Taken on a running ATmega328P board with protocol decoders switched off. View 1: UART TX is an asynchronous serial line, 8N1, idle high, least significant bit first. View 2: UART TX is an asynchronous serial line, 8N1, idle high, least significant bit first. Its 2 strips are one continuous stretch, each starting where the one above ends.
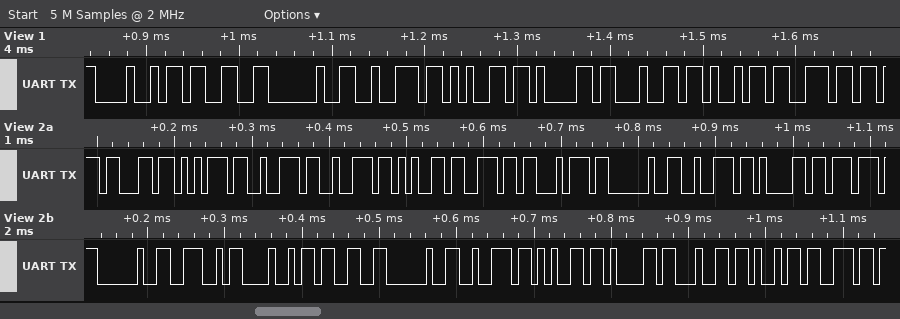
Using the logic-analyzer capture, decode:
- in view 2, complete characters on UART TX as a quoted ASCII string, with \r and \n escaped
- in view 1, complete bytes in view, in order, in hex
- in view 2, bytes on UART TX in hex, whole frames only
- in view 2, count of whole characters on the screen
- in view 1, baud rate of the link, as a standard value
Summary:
"current raw NH3 readin"
48 33 20 72 65 61 64 69 6E
0x63 0x75 0x72 0x72 0x65 0x6E 0x74 0x20 0x72 0x61 0x77 0x20 0x4E 0x48 0x33 0x20 0x72 0x65 0x61 0x64 0x69 0x6E
22
115200 baud
